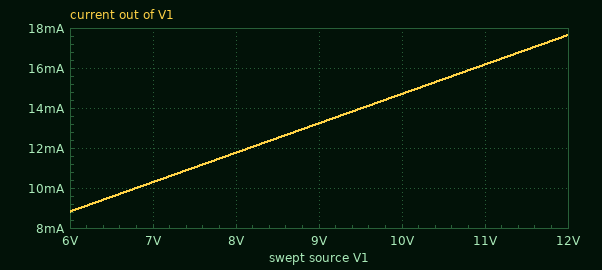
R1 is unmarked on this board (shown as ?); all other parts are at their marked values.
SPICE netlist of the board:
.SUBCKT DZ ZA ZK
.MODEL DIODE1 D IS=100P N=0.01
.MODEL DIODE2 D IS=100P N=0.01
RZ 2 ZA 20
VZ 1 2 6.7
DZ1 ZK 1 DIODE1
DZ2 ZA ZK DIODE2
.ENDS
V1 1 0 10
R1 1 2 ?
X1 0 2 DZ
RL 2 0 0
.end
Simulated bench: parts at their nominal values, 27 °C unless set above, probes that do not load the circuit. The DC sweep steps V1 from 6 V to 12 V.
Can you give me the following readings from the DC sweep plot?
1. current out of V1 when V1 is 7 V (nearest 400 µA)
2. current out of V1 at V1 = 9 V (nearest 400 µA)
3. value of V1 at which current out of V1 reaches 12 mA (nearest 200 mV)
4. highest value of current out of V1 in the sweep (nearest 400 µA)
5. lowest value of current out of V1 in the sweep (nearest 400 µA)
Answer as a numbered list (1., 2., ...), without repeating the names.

1. 10.4 mA
2. 13.2 mA
3. 8.2 V
4. 17.6 mA
5. 8.8 mA
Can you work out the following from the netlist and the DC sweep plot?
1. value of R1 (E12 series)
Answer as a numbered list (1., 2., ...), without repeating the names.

1. 680 Ω
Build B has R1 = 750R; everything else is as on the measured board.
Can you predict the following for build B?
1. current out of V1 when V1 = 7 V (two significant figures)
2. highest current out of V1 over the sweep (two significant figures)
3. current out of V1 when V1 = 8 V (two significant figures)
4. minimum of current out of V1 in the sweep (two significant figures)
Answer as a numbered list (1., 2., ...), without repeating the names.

1. 9.3 mA
2. 16 mA
3. 11 mA
4. 8.0 mA
